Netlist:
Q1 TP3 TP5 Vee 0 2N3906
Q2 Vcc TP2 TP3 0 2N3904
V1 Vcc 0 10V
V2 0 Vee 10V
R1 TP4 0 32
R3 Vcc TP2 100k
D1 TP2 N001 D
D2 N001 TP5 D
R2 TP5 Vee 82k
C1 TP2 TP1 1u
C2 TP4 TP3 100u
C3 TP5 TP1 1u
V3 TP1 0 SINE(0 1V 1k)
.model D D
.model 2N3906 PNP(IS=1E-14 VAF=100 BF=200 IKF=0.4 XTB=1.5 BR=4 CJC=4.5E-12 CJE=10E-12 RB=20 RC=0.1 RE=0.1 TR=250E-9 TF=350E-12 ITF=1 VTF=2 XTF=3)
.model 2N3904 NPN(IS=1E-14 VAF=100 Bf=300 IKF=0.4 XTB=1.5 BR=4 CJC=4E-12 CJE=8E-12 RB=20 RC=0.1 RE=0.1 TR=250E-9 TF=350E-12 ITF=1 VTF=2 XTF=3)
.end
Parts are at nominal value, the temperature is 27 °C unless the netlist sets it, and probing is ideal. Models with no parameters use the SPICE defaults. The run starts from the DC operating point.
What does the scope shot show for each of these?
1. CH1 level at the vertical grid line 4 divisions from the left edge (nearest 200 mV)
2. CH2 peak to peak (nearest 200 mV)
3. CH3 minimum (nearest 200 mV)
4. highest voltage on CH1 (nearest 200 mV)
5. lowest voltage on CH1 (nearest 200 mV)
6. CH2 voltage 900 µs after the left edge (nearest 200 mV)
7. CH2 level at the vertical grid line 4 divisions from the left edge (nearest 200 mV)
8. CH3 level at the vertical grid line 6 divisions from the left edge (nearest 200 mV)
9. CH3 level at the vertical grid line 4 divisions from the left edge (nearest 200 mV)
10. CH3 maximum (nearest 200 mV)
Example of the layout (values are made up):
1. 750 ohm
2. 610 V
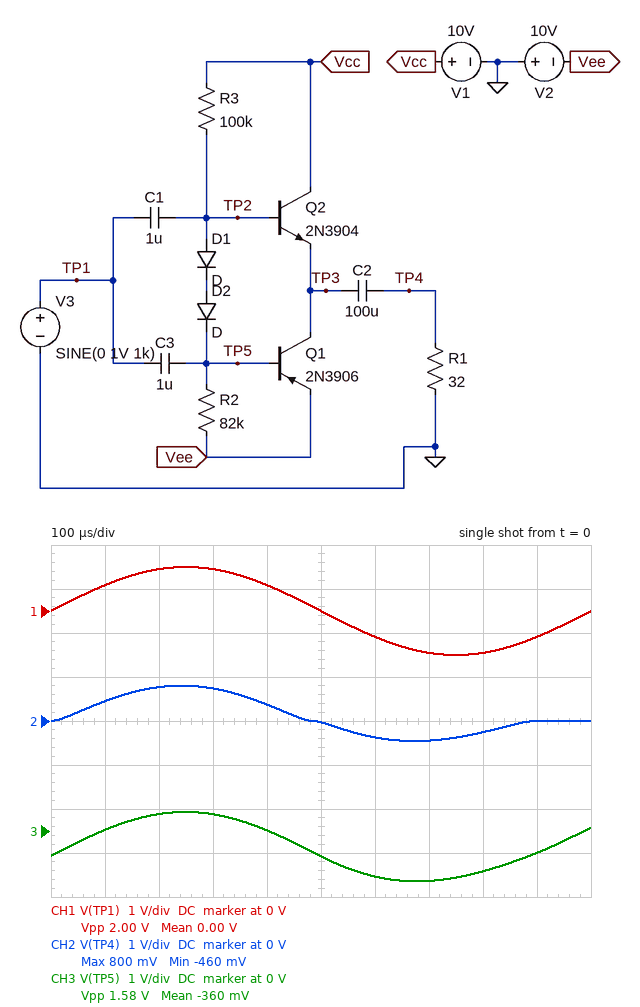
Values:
1. 600 mV
2. 1.2 V
3. -1.2 V
4. 1.0 V
5. -1.0 V
6. 0 V
7. 400 mV
8. -1.0 V
9. 0 V
10. 400 mV
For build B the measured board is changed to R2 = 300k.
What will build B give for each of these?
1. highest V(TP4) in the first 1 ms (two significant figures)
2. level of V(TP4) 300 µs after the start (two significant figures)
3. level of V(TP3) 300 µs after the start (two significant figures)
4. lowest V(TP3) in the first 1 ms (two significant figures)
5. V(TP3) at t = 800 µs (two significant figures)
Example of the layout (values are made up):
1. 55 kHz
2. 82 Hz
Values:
1. 780 mV
2. 720 mV
3. 6.2 V
4. 5.0 V
5. 5.2 V
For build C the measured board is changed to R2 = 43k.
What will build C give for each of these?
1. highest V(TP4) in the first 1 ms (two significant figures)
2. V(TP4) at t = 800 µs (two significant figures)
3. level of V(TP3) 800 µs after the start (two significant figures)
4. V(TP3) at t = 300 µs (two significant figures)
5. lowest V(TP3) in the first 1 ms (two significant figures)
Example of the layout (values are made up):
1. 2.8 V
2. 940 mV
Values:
1. 810 mV
2. -260 mV
3. -3.1 V
4. -2.1 V
5. -3.3 V
